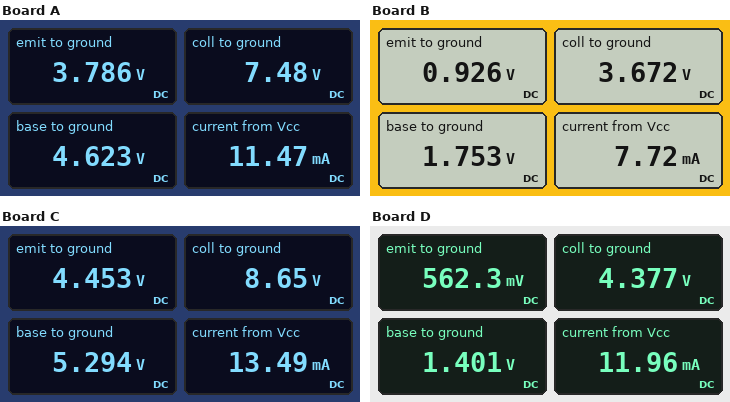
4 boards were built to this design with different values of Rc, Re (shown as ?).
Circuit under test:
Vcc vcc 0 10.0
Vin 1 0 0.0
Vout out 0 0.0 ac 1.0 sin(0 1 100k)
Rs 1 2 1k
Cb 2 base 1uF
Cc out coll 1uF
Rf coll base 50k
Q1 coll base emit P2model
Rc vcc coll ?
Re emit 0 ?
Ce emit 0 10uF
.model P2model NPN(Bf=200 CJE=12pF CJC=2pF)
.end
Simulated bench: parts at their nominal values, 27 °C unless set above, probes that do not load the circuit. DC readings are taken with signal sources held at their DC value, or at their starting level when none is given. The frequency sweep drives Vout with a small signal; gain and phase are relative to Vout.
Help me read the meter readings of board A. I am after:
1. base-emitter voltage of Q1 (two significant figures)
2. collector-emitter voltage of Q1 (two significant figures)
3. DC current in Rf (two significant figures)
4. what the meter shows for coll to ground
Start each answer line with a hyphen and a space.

- 840 mV
- 3.7 V
- 57 µA
- 7.48 V
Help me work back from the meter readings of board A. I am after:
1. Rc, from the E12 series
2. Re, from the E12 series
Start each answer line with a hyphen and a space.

- 220 Ω
- 330 Ω
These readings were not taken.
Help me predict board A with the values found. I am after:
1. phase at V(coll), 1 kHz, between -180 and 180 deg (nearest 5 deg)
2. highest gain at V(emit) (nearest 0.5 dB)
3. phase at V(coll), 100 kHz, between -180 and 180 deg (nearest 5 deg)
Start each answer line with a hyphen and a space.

- 35 deg
- -38.0 dB
- 0 deg
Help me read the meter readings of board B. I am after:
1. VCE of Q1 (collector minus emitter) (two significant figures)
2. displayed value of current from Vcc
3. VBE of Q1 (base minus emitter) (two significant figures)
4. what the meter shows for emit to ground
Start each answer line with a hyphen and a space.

- 2.7 V
- 7.72 mA
- 830 mV
- 0.926 V
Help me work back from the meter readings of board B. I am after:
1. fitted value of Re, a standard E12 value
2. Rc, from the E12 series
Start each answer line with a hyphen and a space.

- 120 Ω
- 820 Ω
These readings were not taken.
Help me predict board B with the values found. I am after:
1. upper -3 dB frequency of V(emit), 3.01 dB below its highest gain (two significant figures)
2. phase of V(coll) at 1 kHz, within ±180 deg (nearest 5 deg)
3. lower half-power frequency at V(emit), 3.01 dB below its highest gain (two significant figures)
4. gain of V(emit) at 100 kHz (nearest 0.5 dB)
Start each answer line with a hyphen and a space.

- 2.7 kHz
- 15 deg
- 34 Hz
- -68.5 dB
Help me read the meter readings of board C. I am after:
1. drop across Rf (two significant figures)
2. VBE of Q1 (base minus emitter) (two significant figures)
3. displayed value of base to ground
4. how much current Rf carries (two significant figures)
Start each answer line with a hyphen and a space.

- 3.4 V
- 840 mV
- 5.294 V
- 67 µA
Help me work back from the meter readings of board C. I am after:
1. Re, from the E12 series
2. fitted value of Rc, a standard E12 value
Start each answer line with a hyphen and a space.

- 330 Ω
- 100 Ω
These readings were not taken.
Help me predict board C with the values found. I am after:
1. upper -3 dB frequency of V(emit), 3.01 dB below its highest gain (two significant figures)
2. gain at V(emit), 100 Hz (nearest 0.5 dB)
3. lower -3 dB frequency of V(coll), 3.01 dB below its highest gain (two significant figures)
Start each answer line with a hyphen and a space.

- 5.3 kHz
- -53.5 dB
- 2.0 kHz
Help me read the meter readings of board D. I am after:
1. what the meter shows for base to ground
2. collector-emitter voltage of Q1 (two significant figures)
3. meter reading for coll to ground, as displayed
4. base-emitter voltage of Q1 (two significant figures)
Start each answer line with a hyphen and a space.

- 1.401 V
- 3.8 V
- 4.377 V
- 840 mV
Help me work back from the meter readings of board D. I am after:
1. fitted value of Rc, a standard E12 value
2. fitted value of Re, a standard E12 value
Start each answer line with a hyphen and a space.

- 470 Ω
- 47 Ω
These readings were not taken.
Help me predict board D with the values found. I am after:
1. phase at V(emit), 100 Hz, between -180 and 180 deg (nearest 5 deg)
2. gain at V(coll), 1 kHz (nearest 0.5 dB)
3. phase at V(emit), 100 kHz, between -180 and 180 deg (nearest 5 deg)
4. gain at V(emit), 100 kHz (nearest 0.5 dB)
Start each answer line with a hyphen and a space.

- 35 deg
- -1.5 dB
- -85 deg
- -67.0 dB
